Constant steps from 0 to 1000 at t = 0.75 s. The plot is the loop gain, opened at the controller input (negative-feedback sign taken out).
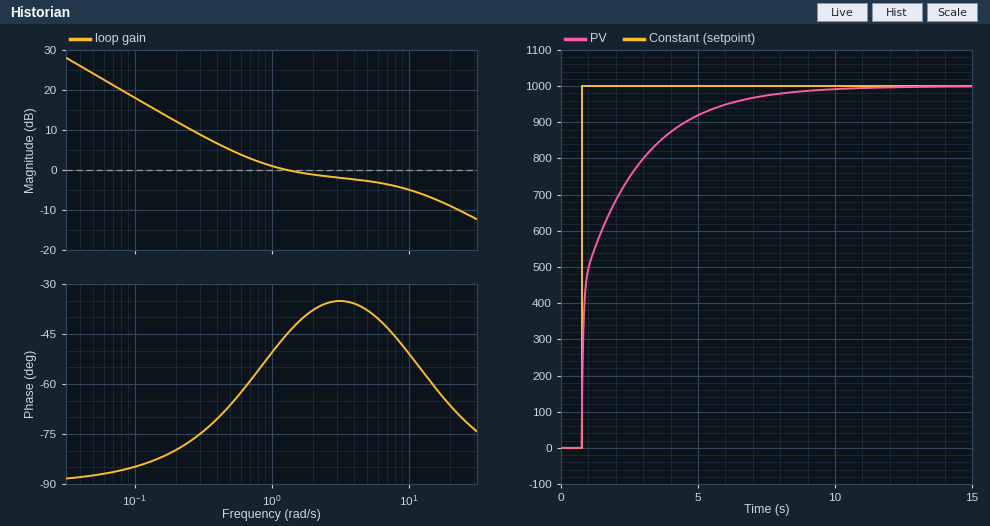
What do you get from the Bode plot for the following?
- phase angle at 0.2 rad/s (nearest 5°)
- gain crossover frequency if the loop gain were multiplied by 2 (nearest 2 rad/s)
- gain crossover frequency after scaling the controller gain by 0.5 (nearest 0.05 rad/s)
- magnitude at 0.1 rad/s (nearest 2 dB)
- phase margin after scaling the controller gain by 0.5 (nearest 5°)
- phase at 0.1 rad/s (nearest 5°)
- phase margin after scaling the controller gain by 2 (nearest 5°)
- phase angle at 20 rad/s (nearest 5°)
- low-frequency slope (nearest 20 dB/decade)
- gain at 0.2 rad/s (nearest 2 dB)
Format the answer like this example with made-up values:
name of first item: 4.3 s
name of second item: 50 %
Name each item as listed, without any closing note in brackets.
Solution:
phase angle at 0.2 rad/s: -80°
gain crossover frequency if the loop gain were multiplied by 2: 12 rad/s
gain crossover frequency after scaling the controller gain by 0.5: 0.45 rad/s
magnitude at 0.1 rad/s: 18 dB
phase margin after scaling the controller gain by 0.5: 110°
phase at 0.1 rad/s: -85°
phase margin after scaling the controller gain by 2: 125°
phase angle at 20 rad/s: -65°
low-frequency slope: -20 dB/decade
gain at 0.2 rad/s: 12 dB
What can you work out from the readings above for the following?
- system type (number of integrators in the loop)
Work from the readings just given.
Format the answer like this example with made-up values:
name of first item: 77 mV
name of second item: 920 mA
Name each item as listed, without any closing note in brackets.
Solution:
system type: 1
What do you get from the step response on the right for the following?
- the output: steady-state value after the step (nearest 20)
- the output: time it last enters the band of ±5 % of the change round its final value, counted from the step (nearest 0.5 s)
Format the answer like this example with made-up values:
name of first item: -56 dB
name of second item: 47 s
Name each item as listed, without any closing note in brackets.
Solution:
the output: steady-state value after the step: 1000
the output: time it last enters the band of ±5 % of the change round its final value, counted from the step: 5.5 s
